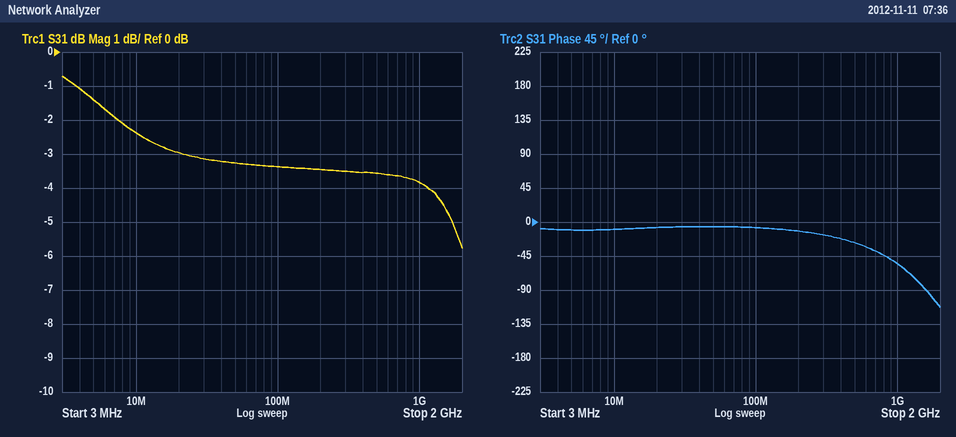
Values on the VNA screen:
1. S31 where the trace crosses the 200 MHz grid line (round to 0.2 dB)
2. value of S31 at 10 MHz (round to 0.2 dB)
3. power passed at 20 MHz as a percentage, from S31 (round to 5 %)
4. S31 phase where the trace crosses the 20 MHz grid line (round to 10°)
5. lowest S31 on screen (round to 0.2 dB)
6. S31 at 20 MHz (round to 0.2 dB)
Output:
-3.4 dB
-2.4 dB
50 %
-10°
-5.8 dB
-3.0 dB
